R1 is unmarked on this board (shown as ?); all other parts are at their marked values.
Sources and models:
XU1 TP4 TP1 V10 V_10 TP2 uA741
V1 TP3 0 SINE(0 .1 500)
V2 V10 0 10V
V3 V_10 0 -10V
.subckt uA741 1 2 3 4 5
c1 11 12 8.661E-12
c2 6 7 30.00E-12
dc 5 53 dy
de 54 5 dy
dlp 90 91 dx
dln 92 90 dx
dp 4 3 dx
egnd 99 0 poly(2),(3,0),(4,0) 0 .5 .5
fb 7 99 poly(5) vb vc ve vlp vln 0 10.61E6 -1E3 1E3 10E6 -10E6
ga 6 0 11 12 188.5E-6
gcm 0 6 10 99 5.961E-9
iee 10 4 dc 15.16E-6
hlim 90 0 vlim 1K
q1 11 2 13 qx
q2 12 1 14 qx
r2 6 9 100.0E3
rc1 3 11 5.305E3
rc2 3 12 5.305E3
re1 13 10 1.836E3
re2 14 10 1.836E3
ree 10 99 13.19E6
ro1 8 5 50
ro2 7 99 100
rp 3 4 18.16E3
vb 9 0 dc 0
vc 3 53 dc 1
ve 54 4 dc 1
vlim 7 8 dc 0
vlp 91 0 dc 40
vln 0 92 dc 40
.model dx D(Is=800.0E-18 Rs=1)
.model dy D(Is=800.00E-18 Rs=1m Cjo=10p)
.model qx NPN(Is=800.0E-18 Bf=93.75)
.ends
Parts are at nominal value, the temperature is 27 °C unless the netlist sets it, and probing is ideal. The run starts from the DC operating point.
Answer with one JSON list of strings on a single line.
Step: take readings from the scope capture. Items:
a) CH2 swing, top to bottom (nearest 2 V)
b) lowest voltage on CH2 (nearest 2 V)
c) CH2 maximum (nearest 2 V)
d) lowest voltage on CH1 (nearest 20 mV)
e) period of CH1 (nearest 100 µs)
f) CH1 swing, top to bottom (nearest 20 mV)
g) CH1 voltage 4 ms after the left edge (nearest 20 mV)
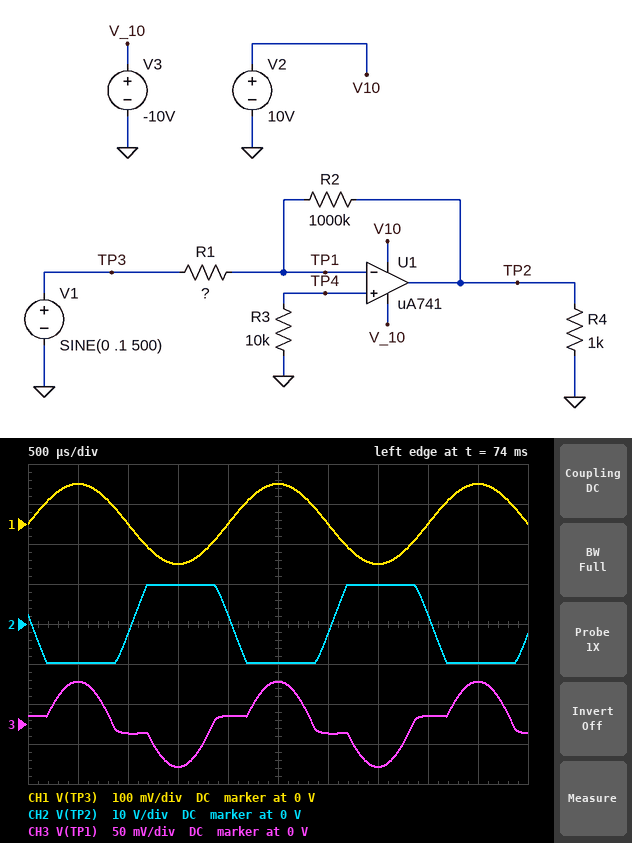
["20 V", "-10 V", "10 V", "-100 mV", "2.0 ms", "200 mV", "0 V"]
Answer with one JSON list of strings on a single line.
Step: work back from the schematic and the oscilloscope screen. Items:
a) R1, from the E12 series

["4.7 kΩ"]
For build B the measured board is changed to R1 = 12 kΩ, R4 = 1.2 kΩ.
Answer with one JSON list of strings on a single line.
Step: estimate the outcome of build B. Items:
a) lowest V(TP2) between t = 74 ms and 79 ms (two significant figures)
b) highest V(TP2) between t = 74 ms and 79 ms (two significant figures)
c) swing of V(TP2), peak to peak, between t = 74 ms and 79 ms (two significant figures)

["-8.3 V", "8.3 V", "17 V"]
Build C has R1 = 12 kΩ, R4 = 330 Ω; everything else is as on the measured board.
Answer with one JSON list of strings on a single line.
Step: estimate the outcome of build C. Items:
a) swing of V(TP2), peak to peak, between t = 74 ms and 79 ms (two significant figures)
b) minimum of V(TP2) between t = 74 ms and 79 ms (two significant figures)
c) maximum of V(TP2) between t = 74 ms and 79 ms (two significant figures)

["17 V", "-8.3 V", "8.3 V"]
